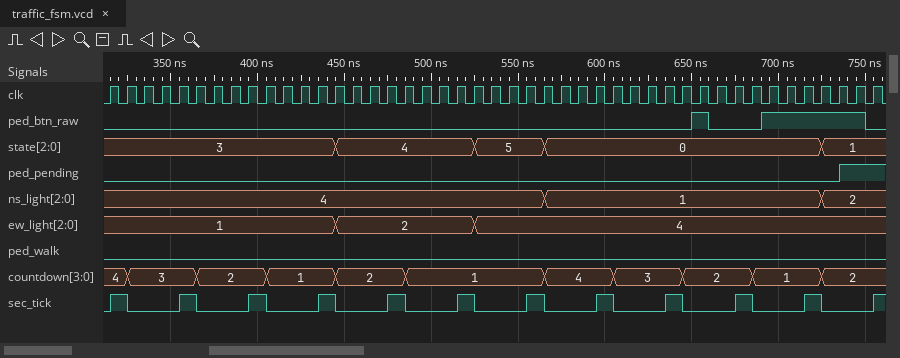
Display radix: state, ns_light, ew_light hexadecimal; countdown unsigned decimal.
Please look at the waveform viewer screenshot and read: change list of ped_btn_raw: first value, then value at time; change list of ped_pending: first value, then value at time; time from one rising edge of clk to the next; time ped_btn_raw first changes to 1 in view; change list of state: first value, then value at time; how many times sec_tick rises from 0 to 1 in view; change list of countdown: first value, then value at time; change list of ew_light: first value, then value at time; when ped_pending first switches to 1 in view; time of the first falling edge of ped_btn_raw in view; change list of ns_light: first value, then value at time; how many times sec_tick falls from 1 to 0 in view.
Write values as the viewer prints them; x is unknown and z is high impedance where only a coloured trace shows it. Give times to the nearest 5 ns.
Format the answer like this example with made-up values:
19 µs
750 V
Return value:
0, 1 at 650 ns, 0 at 660 ns, 1 at 690 ns, 0 at 750 ns
0, 1 at 735 ns
10 ns
650 ns
3, 4 at 445 ns, 5 at 525 ns, 0 at 565 ns, 1 at 725 ns
12
4, 3 at 325 ns, 2 at 365 ns, 1 at 405 ns, 2 at 445 ns, 1 at 485 ns, 4 at 565 ns, 3 at 605 ns, 2 at 645 ns, 1 at 685 ns, 2 at 725 ns
1, 2 at 445 ns, 4 at 525 ns
735 ns
660 ns
4, 1 at 565 ns, 2 at 725 ns
11
